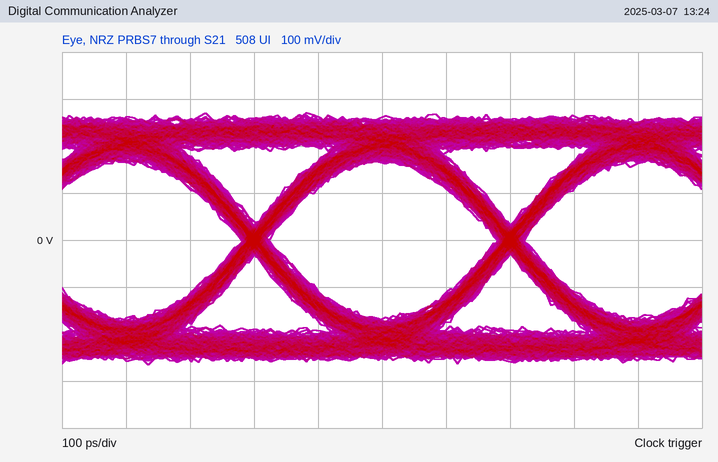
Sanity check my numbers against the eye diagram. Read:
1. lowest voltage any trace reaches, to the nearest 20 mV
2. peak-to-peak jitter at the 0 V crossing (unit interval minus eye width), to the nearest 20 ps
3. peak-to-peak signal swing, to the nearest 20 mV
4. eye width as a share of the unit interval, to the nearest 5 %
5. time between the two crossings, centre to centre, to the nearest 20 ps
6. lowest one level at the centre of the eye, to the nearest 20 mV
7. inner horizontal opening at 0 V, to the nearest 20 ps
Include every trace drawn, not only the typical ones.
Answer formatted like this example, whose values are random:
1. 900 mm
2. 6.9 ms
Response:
1. -260 mV
2. 40 ps
3. 540 mV
4. 90 %
5. 400 ps
6. 160 mV
7. 360 ps
